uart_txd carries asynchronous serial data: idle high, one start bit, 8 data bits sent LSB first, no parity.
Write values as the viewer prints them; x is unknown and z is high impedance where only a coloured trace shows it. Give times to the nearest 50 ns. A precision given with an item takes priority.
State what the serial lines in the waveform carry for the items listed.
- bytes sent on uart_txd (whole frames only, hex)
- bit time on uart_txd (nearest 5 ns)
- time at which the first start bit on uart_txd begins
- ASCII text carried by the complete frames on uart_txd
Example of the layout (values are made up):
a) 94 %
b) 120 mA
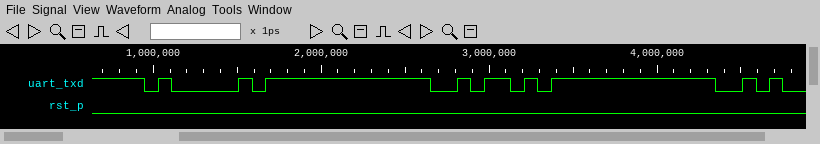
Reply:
a) 41, 5A
b) 80 ns
c) 950 ns
d) "AZ"
